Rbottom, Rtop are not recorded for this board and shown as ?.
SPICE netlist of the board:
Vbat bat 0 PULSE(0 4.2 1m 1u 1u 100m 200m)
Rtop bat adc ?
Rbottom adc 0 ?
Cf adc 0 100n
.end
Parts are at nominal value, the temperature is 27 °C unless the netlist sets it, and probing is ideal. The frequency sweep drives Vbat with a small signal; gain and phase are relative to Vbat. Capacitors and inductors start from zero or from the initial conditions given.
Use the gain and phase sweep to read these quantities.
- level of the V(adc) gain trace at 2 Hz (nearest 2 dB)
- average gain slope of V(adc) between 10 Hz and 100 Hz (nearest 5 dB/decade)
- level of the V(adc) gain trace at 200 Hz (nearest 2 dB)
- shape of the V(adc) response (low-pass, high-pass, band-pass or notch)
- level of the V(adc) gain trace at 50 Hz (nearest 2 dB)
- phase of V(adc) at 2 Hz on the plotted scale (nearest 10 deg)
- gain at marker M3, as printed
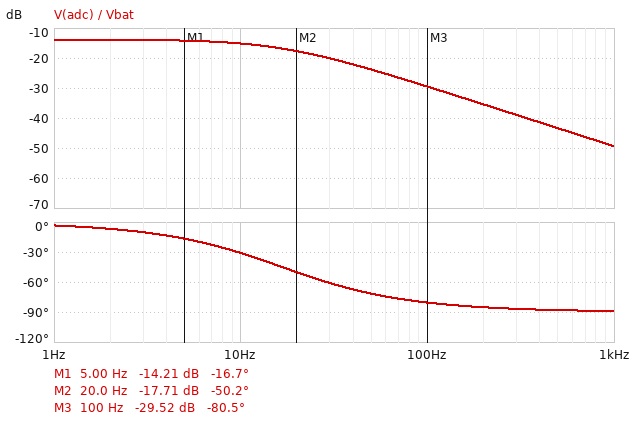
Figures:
-14 dB
-15 dB/decade
-36 dB
low-pass
-24 dB
-10 deg
-29.52 dB
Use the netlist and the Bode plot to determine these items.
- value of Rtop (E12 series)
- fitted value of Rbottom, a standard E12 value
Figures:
470 kΩ
120 kΩ
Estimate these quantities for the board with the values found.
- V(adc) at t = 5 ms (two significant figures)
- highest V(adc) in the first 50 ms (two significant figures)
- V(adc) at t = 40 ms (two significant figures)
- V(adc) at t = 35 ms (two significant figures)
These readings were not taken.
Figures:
290 mV
850 mV
840 mV
830 mV
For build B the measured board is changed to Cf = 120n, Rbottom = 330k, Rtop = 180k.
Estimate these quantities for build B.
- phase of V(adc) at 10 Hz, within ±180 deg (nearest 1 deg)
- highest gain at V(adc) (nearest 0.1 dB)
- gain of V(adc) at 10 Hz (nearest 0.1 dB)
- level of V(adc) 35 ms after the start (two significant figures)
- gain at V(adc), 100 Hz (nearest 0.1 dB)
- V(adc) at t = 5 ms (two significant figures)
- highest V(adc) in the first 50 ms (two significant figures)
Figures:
-41 deg
-3.8 dB
-6.3 dB
2.5 V
-22.7 dB
680 mV
2.6 V
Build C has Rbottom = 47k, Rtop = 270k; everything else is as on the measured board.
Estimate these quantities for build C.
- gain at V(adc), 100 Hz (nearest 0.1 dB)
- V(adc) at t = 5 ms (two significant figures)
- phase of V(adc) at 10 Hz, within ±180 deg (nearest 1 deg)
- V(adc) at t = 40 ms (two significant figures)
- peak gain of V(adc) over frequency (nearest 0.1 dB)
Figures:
-25.2 dB
390 mV
-14 deg
620 mV
-16.6 dB
